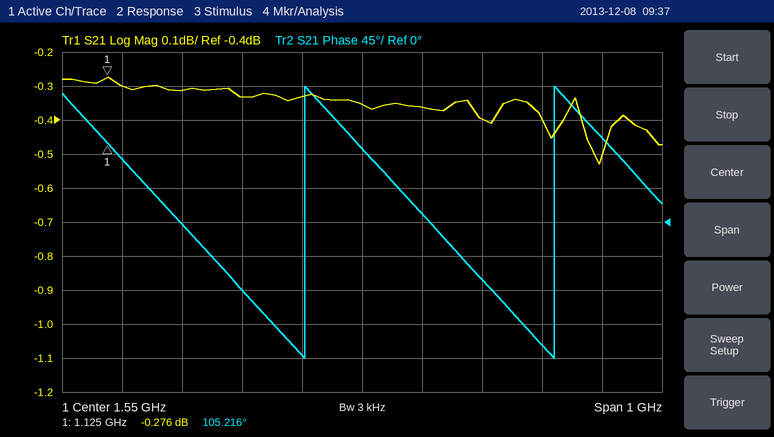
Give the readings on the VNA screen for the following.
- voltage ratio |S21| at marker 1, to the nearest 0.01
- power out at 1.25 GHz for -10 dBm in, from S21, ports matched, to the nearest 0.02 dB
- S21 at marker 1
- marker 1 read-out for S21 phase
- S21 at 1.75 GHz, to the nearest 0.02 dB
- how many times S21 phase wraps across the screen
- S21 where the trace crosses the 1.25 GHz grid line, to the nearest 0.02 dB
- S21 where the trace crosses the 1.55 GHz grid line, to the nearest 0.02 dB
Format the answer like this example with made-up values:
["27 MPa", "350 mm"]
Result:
["0.97", "-10.32 dBm", "-0.276 dB", "105.216°", "-0.40 dB", "2", "-0.32 dB", "-0.36 dB"]
